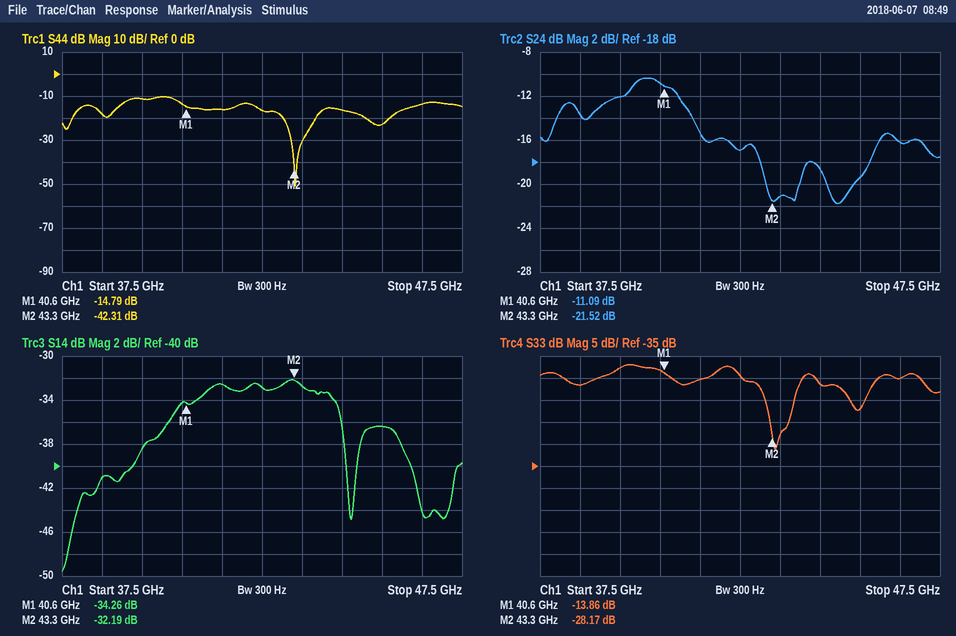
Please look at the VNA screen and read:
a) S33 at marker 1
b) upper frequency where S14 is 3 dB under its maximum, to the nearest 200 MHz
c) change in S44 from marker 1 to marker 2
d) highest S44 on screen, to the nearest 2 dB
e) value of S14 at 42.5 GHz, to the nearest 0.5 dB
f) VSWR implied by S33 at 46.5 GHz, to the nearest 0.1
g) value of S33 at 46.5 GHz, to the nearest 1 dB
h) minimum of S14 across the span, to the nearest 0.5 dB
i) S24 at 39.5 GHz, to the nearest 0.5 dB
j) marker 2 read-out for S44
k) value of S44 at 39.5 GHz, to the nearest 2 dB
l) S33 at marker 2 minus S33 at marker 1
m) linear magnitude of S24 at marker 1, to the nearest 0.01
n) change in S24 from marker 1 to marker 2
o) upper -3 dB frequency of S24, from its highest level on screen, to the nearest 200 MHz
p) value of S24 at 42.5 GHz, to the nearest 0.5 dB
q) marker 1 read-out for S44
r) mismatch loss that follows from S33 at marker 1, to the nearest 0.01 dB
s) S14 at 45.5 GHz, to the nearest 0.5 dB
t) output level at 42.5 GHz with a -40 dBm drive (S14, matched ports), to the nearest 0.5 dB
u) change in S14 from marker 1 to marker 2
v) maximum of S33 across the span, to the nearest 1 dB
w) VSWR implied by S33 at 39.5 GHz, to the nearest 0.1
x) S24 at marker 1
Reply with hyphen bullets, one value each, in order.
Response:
- -13.86 dB
- 44.4 GHz
- -27.52 dB
- -10 dB
- -33.0 dB
- 1.4
- -15 dB
- -49.5 dB
- -12.0 dB
- -42.31 dB
- -12 dB
- -14.31 dB
- 0.28
- -10.43 dB
- 41.2 GHz
- -17.0 dB
- -14.79 dB
- 0.18 dB
- -36.5 dB
- -73.0 dBm
- 2.07 dB
- -12 dB
- 1.6
- -11.09 dB
